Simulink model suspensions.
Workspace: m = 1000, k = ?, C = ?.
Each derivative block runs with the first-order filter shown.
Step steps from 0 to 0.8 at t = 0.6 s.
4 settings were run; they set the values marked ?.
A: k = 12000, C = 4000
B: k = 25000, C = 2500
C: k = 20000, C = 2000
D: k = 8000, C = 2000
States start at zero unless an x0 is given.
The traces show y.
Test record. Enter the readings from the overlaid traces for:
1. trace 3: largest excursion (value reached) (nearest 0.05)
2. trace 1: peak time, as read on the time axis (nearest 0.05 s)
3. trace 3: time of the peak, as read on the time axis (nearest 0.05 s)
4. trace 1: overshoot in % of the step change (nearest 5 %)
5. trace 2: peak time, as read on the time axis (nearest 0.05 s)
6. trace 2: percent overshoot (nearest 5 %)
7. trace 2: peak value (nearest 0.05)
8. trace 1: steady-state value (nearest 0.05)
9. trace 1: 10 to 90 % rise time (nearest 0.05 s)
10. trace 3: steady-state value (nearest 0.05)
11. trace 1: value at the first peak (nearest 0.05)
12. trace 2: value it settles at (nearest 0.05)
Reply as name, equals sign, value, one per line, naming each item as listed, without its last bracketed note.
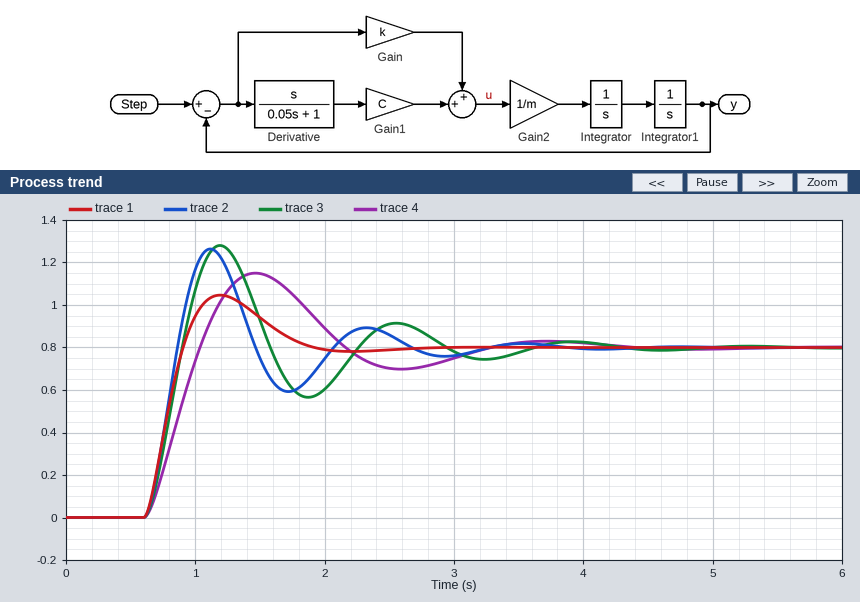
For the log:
trace 3: largest excursion (value reached) = 1.30
trace 1: peak time, as read on the time axis = 1.20 s
trace 3: time of the peak, as read on the time axis = 1.20 s
trace 1: overshoot in % of the step change = 30 %
trace 2: peak time, as read on the time axis = 1.10 s
trace 2: percent overshoot = 60 %
trace 2: peak value = 1.25
trace 1: steady-state value = 0.80
trace 1: 10 to 90 % rise time = 0.20 s
trace 3: steady-state value = 0.80
trace 1: value at the first peak = 1.05
trace 2: value it settles at = 0.80
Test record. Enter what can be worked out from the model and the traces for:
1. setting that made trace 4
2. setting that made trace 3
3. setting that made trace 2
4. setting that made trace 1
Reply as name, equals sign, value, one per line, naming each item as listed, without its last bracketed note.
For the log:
setting that made trace 4 = D
setting that made trace 3 = C
setting that made trace 2 = B
setting that made trace 1 = A
